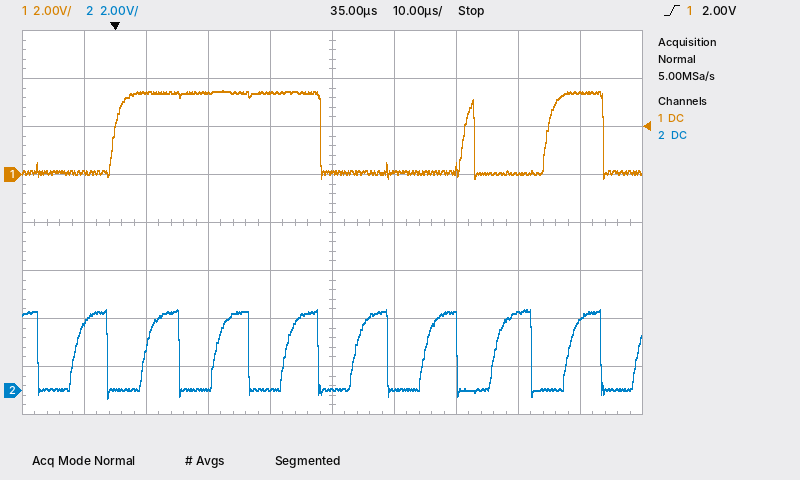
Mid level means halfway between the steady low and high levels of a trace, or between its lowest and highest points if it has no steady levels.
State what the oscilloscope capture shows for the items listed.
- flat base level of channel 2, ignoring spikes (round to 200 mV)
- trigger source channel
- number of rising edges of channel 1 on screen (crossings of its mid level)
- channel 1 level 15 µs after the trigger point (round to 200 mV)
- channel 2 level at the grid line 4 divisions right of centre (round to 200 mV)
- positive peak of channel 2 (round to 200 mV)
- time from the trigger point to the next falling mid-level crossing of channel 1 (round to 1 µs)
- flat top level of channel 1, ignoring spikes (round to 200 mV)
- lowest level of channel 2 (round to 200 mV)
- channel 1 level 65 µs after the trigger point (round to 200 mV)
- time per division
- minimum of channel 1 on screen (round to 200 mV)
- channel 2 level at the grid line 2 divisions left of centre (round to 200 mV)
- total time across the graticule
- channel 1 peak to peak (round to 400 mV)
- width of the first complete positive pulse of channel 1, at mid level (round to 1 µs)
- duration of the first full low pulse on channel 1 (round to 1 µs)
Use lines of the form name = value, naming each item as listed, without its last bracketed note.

flat base level of channel 2, ignoring spikes = 0.0 V
trigger source channel = channel 1
number of rising edges of channel 1 on screen = 3
channel 1 level 15 µs after the trigger point = 3.4 V
channel 2 level at the grid line 4 divisions right of centre = 3.0 V
positive peak of channel 2 = 3.4 V
time from the trigger point to the next falling mid-level crossing of channel 1 = 33 µs
flat top level of channel 1, ignoring spikes = 3.4 V
lowest level of channel 2 = -400 mV
channel 1 level 65 µs after the trigger point = 0.0 V
time per division = 10 µs
minimum of channel 1 on screen = -200 mV
channel 2 level at the grid line 2 divisions left of centre = 0.0 V
total time across the graticule = 100 µs
channel 1 peak to peak = 3.6 V
width of the first complete positive pulse of channel 1, at mid level = 33 µs
duration of the first full low pulse on channel 1 = 23 µs
